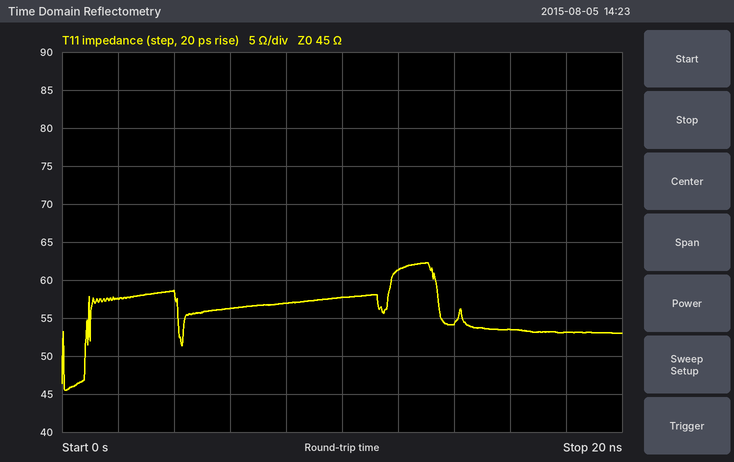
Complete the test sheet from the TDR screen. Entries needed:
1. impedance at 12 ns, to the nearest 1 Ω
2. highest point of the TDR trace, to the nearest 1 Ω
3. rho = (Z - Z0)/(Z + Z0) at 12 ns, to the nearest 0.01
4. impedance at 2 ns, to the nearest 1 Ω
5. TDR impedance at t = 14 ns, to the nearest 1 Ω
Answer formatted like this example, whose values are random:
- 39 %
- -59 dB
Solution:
- 61 Ω
- 62 Ω
- +0.15
- 58 Ω
- 54 Ω
